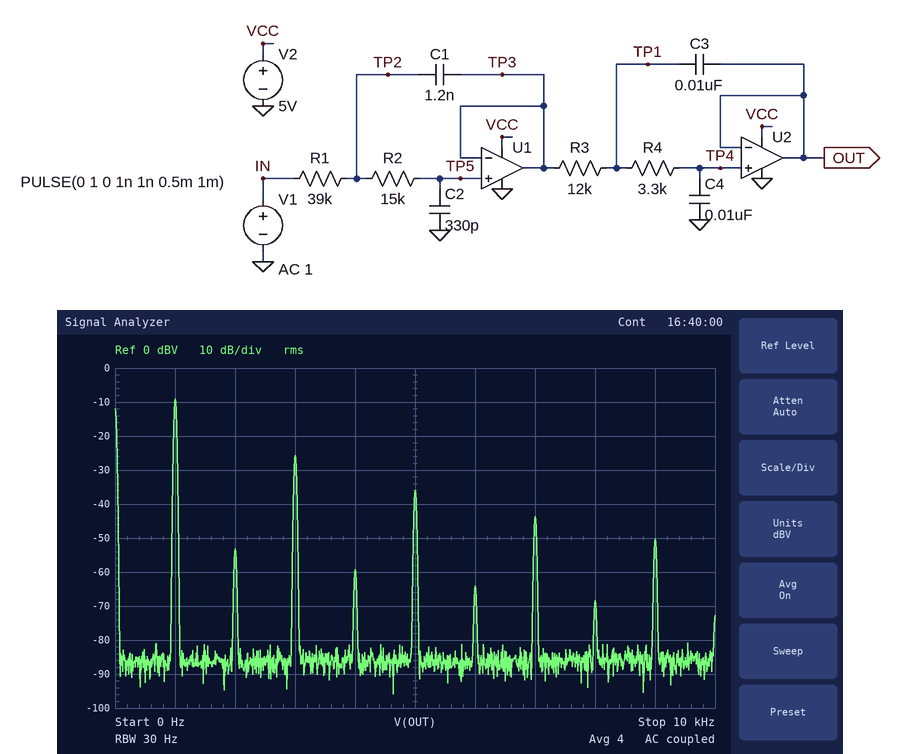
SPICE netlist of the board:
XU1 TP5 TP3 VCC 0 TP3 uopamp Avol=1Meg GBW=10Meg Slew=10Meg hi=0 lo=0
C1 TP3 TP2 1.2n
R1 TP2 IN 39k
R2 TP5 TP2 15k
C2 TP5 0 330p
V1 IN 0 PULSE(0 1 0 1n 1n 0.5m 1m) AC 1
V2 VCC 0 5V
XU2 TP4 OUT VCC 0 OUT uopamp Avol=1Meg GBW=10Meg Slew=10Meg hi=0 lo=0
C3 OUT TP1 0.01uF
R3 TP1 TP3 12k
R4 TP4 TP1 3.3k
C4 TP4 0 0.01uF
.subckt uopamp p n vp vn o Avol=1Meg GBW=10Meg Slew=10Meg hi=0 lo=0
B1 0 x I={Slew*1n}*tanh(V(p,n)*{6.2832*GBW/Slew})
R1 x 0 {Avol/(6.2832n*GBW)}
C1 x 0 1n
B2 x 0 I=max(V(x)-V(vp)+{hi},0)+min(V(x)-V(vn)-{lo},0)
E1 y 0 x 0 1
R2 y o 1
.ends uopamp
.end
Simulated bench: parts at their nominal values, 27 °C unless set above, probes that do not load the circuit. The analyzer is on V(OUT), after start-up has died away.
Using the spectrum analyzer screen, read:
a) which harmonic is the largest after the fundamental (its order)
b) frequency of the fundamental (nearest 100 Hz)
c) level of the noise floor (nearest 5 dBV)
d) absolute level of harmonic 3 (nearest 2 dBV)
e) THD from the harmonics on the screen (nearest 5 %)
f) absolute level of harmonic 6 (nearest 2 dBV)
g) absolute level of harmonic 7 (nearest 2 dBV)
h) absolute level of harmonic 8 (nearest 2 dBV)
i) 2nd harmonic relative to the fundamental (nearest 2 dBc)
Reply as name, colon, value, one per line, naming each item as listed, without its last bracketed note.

which harmonic is the largest after the fundamental: 3
frequency of the fundamental: 1.0 kHz
level of the noise floor: -85 dBV
absolute level of harmonic 3: -26 dBV
THD from the harmonics on the screen: 15 %
absolute level of harmonic 6: -64 dBV
absolute level of harmonic 7: -44 dBV
absolute level of harmonic 8: -68 dBV
2nd harmonic relative to the fundamental: -44 dBc
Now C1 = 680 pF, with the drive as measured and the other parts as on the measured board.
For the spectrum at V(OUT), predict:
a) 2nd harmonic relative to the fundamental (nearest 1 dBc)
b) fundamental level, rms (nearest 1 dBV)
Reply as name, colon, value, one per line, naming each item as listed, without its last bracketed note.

2nd harmonic relative to the fundamental: -59 dBc
fundamental level, rms: -9 dBV
